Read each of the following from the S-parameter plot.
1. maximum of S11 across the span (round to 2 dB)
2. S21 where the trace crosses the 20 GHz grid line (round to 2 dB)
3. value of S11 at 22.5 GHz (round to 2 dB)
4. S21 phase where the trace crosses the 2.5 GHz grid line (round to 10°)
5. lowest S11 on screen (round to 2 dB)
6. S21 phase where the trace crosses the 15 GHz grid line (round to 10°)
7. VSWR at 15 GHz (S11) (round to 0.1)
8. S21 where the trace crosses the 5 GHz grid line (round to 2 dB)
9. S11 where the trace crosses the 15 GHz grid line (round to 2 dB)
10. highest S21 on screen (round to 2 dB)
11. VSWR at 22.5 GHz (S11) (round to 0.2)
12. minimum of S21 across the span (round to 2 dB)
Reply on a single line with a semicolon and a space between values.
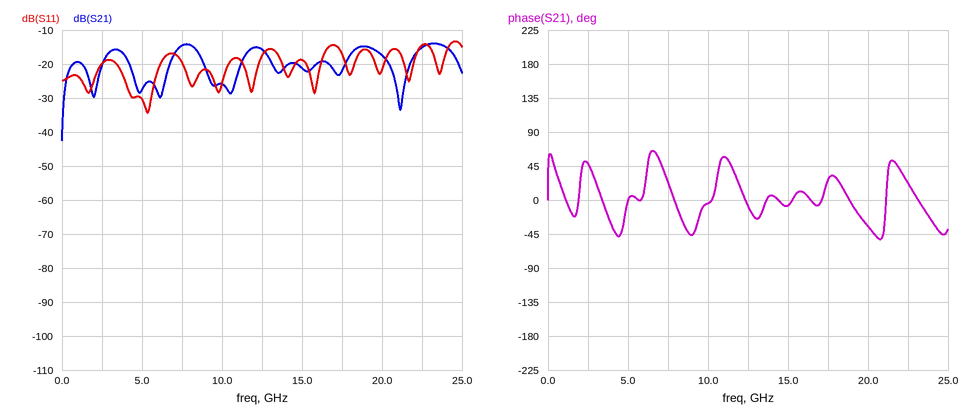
-14 dB; -18 dB; -14 dB; 50°; -34 dB; -10°; 1.3; -28 dB; -18 dB; -14 dB; 1.4; -42 dB
